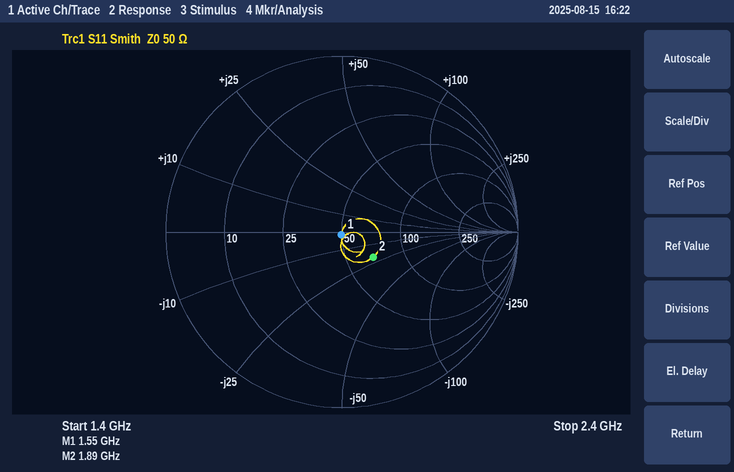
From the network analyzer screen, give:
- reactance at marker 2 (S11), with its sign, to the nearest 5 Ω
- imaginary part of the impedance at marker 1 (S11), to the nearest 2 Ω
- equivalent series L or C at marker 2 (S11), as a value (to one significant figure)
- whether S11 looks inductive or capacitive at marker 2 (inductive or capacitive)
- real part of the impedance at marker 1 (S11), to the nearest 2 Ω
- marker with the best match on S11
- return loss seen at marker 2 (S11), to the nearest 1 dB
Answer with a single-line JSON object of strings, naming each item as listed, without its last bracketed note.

{"reactance at marker 2 (S11), with its sign, to the nearest 5 Ω": "-20 Ω", "imaginary part of the impedance at marker 1 (S11), to the nearest 2 Ω": "-2 Ω", "equivalent series L or C at marker 2 (S11), as a value": "4 pF", "whether S11 looks inductive or capacitive at marker 2": "capacitive", "real part of the impedance at marker 1 (S11), to the nearest 2 Ω": "50 Ω", "marker with the best match on S11": "marker 1", "return loss seen at marker 2 (S11), to the nearest 1 dB": "13 dB"}
